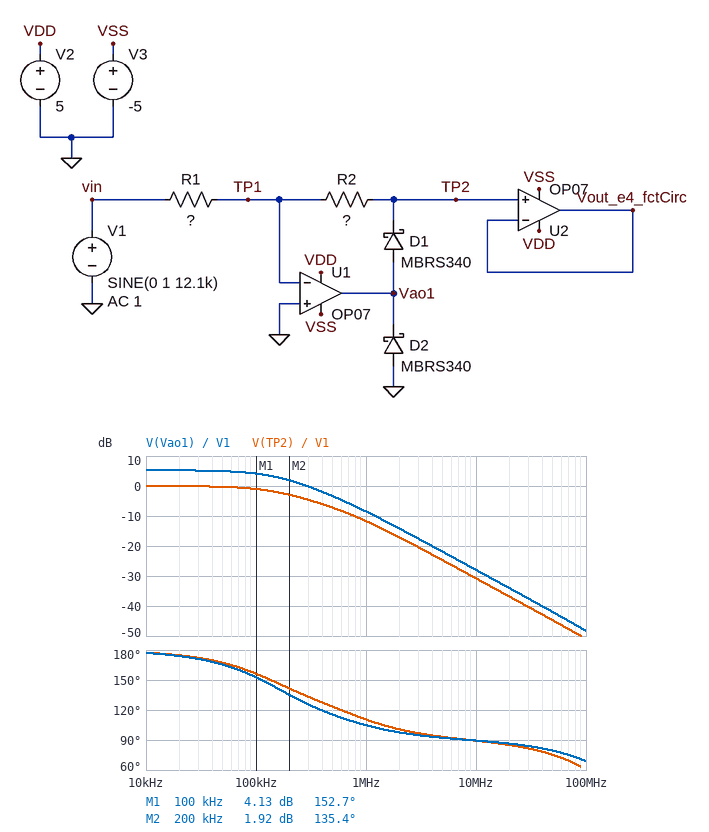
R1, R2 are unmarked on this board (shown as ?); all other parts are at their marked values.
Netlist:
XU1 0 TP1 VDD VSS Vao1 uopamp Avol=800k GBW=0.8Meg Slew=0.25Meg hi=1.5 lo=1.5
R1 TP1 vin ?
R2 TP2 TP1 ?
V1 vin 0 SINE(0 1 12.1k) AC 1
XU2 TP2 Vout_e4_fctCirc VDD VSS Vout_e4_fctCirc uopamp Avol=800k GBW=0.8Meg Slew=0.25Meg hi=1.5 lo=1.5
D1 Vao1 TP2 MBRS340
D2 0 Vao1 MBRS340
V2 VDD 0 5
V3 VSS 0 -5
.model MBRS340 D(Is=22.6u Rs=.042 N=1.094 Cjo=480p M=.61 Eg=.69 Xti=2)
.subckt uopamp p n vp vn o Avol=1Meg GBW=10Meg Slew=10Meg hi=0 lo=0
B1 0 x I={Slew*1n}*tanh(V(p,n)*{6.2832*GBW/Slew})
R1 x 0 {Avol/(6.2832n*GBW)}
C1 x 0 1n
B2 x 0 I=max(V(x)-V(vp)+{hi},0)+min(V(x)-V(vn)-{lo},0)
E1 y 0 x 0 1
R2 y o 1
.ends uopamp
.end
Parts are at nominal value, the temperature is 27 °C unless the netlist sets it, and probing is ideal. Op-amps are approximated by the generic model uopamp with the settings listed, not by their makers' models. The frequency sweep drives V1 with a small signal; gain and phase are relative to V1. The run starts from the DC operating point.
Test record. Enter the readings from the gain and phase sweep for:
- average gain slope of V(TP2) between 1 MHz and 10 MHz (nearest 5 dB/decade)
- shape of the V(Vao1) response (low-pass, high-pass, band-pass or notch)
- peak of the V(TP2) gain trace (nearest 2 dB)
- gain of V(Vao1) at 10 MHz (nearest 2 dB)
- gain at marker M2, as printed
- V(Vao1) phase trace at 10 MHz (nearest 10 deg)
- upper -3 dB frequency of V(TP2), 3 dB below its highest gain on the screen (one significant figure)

-20 dB/decade
low-pass
0 dB
-28 dB
1.92 dB
90 deg
200 kHz
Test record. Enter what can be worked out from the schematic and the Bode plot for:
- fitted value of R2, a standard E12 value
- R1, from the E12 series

1.5 kΩ
1.5 kΩ
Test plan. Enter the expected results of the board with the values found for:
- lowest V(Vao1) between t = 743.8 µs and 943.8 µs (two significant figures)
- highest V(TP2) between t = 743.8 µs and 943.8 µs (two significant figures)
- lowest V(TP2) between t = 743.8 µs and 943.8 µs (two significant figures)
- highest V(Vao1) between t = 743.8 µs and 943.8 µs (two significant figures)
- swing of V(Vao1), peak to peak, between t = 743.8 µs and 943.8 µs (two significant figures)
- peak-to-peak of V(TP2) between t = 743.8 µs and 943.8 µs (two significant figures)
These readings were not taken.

-460 mV
1.0 V
-400 mV
1.1 V
1.6 V
1.4 V
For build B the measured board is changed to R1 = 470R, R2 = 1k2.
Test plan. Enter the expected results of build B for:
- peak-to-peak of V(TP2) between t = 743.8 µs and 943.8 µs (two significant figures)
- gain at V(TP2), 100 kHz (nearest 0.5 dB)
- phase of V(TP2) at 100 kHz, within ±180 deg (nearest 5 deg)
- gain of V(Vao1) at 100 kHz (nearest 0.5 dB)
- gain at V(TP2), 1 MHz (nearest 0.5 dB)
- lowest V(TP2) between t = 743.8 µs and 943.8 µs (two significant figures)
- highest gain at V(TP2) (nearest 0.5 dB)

2.8 V
5.5 dB
140 deg
11.5 dB
-9.0 dB
-410 mV
8.0 dB
